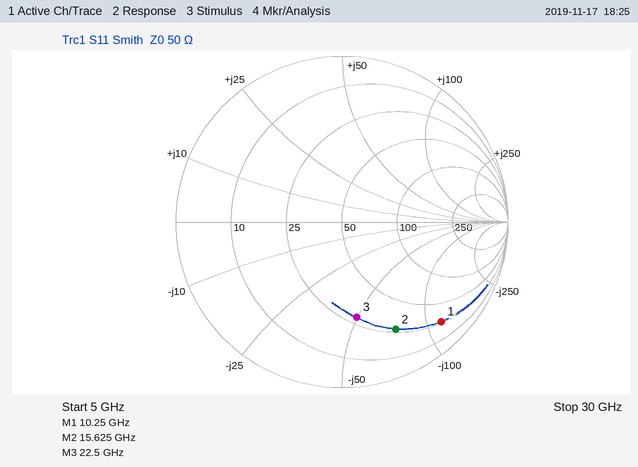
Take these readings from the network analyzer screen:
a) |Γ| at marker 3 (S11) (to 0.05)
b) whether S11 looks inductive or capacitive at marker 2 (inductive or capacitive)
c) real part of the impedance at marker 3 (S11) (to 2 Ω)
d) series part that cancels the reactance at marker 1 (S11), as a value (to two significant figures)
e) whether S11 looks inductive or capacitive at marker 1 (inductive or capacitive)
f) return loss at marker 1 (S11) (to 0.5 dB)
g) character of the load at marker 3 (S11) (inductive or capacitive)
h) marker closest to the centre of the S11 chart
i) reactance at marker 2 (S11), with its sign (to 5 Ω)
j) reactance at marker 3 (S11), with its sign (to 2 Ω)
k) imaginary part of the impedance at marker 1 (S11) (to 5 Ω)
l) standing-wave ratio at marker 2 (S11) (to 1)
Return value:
0.60
capacitive
28 Ω
1.8 nH
capacitive
1.5 dB
capacitive
marker 3
-75 Ω
-50 Ω
-115 Ω
6
